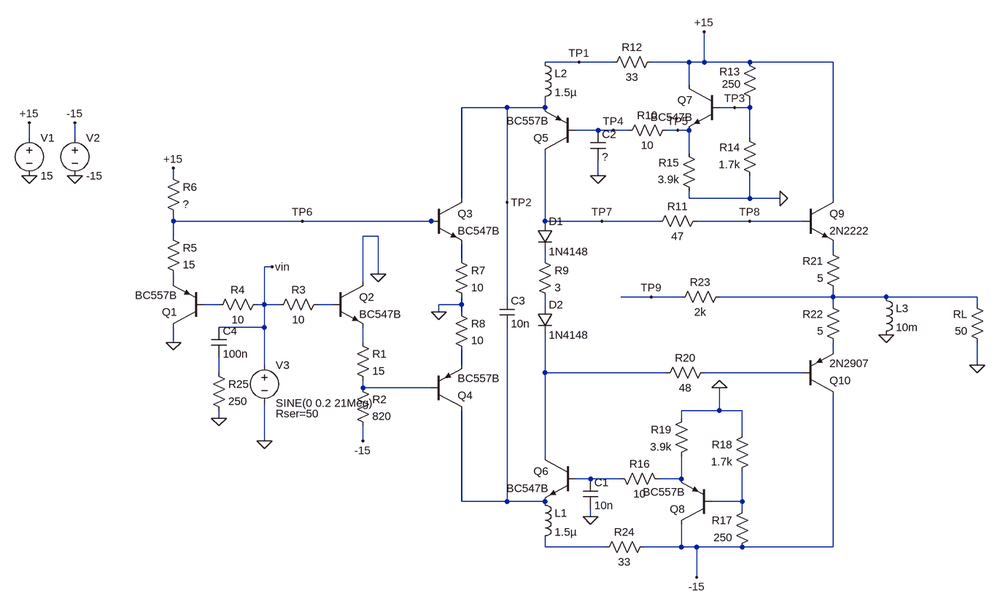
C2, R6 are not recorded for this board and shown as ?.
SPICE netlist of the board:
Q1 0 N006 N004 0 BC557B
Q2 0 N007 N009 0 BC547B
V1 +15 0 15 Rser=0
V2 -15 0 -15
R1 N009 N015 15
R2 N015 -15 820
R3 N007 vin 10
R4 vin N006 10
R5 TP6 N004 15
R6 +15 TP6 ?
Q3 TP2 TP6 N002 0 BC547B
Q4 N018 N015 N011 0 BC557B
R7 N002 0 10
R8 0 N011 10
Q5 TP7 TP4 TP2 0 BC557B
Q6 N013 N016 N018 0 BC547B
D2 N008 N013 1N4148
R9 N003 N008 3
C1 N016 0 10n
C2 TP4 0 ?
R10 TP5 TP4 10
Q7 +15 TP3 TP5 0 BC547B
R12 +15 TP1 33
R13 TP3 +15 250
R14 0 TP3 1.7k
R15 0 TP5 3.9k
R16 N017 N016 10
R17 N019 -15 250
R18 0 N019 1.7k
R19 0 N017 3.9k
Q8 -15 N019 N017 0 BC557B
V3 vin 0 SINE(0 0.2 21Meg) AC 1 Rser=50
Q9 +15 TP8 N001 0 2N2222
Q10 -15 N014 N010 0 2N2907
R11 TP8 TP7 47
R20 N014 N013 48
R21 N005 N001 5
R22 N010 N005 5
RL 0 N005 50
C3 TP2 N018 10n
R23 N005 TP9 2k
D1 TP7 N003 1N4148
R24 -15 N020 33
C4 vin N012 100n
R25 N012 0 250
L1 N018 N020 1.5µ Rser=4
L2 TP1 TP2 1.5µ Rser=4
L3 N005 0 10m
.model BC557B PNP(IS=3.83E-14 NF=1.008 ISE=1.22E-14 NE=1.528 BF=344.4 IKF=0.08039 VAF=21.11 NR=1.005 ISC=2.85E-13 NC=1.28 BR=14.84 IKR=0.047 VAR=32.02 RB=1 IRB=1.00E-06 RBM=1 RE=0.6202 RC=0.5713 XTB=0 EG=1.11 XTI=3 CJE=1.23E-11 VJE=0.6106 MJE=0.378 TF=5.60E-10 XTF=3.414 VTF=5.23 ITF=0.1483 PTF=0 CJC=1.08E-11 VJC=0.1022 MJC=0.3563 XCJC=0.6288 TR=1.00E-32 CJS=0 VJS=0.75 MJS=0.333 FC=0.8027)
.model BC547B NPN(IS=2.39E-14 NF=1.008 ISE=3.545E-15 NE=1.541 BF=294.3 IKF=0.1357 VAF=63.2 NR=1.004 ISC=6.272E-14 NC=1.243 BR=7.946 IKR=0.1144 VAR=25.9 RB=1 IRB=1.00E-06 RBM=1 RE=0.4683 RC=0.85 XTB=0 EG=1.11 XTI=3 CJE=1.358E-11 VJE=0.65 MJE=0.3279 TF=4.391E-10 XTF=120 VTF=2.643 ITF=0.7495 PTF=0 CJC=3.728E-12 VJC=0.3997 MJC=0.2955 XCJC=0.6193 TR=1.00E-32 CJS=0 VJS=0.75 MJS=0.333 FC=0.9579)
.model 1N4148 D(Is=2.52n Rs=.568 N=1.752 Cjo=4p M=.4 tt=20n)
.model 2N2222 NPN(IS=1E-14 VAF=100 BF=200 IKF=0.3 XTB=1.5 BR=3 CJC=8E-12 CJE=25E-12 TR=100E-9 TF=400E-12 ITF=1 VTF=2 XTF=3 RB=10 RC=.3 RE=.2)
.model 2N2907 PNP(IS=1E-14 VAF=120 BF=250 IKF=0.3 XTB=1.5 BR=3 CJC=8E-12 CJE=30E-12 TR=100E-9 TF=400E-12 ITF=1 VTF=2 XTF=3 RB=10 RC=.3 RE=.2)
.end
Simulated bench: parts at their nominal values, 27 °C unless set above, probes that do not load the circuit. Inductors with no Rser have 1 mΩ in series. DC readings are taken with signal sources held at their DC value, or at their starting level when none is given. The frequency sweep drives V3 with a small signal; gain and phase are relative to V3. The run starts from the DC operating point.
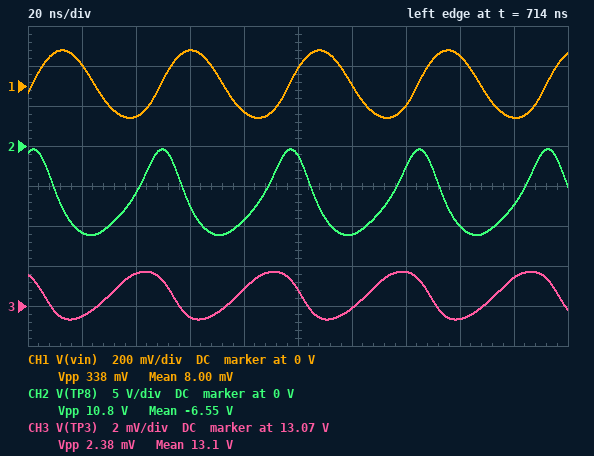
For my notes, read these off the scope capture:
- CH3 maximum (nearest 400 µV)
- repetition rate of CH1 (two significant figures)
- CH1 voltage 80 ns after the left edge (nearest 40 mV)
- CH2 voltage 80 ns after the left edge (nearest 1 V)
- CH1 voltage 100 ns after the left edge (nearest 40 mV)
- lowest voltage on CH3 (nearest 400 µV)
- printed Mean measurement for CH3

13.0756 V
21 MHz
-120 mV
-9 V
80 mV
13.0732 V
13.1 V
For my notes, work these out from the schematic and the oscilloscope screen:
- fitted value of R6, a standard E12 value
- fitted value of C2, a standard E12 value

390 Ω
6.8 nF
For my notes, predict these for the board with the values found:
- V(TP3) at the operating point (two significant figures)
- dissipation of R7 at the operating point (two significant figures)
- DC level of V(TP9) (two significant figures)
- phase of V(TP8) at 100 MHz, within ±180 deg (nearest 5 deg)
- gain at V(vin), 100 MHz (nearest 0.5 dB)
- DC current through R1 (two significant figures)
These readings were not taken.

13 V
26 mW
-1.2 mV
-15 deg
-6.0 dB
17 mA
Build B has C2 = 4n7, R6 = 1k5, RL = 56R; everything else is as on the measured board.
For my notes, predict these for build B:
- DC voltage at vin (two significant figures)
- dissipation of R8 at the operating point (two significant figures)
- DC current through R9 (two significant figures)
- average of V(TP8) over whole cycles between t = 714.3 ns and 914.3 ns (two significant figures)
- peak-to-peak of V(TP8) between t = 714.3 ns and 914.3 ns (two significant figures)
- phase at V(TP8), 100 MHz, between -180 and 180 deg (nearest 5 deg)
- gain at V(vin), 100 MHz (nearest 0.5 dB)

-1.8 mV
6.8 mW
24 mA
4.1 V
15 V
-30 deg
-5.0 dB
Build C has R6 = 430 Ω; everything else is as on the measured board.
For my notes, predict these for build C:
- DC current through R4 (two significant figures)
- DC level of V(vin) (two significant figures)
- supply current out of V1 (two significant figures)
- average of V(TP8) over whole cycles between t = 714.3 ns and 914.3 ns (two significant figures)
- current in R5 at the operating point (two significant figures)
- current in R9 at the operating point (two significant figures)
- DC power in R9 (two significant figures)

130 µA
3.3 mV
95 mA
-5.8 V
32 mA
6.0 mA
110 µW
